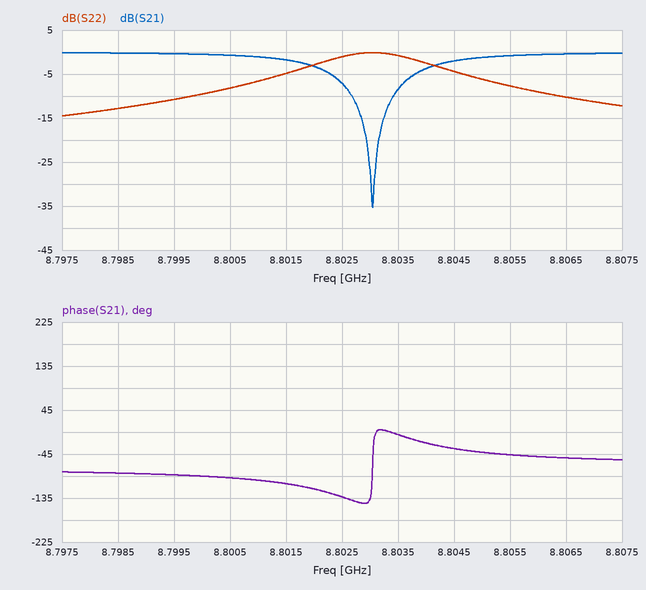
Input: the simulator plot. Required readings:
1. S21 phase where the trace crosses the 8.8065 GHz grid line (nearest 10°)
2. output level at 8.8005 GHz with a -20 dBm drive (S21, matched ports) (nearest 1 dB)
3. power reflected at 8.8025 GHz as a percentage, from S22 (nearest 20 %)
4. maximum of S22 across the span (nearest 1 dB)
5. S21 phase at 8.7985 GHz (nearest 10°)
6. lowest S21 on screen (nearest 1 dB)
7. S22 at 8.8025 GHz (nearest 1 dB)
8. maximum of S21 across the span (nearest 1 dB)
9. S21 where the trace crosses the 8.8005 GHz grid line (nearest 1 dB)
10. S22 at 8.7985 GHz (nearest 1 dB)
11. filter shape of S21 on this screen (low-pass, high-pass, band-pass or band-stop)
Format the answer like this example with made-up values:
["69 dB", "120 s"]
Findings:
["-50°", "-21 dBm", "80 %", "0 dB", "-80°", "-35 dB", "-1 dB", "0 dB", "-1 dB", "-13 dB", "band-stop"]
